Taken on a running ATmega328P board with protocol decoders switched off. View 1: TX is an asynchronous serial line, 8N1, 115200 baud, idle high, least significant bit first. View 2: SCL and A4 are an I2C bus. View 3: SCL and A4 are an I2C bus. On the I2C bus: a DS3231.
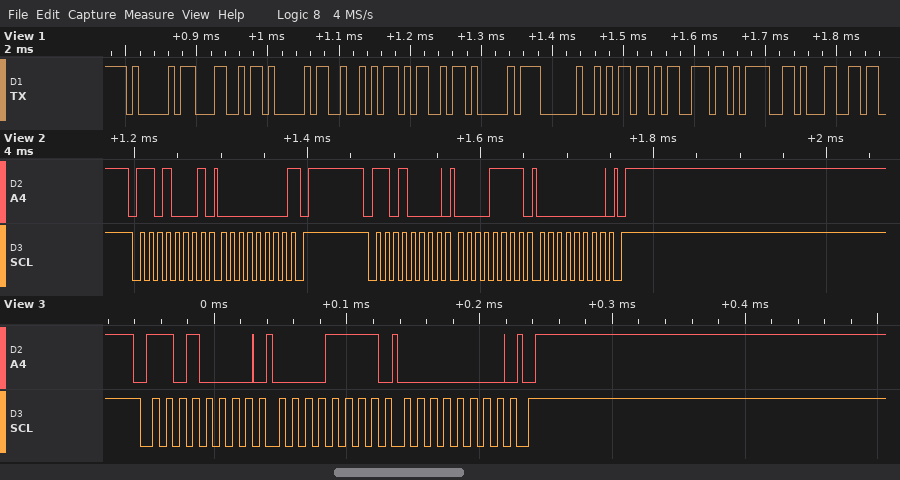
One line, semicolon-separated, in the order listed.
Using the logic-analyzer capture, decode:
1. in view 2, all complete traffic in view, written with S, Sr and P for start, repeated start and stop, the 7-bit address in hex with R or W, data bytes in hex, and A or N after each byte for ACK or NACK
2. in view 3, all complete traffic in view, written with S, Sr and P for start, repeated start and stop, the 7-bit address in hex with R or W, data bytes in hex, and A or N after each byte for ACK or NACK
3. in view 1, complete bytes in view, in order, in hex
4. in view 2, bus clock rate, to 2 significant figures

S 68R A 00 N P S 68W A 0F A 00 A P; S 68W A 0F A 00 A P; 41 4C 41 52 4D 41 20 6D 73 3D 31; 100 kHz
